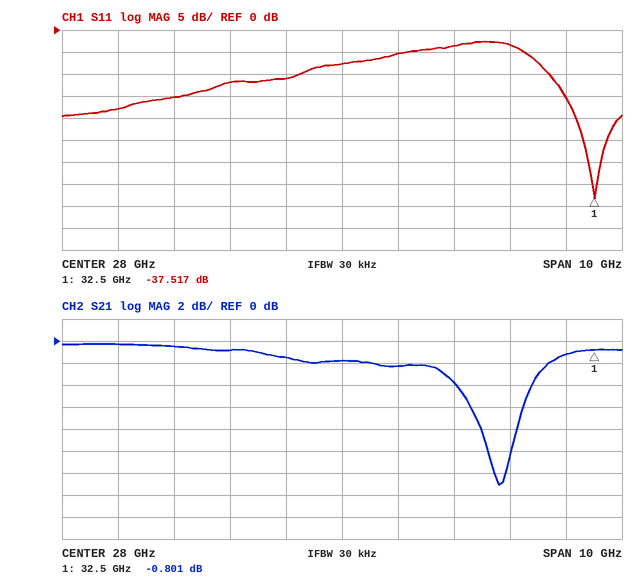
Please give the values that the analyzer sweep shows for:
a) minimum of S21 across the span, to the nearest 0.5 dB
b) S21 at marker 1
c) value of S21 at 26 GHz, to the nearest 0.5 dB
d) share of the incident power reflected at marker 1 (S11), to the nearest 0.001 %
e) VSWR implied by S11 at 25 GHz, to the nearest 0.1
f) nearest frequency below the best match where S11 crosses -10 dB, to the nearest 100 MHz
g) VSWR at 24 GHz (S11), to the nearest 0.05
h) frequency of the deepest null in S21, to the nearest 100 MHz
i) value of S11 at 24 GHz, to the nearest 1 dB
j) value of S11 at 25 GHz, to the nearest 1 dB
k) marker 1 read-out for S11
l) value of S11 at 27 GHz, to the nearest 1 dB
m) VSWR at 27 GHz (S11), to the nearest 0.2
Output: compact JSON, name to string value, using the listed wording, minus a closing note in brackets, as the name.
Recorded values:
{"minimum of S21 across the span, to the nearest 0.5 dB": "-13.0 dB", "S21 at marker 1": "-0.801 dB", "value of S21 at 26 GHz, to the nearest 0.5 dB": "-1.0 dB", "share of the incident power reflected at marker 1 (S11), to the nearest 0.001 %": "0.018 %", "VSWR implied by S11 at 25 GHz, to the nearest 0.1": "1.4", "nearest frequency below the best match where S11 crosses -10 dB, to the nearest 100 MHz": "31.7 GHz", "VSWR at 24 GHz (S11), to the nearest 0.05": "1.30", "frequency of the deepest null in S21, to the nearest 100 MHz": "30.8 GHz", "value of S11 at 24 GHz, to the nearest 1 dB": "-18 dB", "value of S11 at 25 GHz, to the nearest 1 dB": "-15 dB", "marker 1 read-out for S11": "-37.517 dB", "value of S11 at 27 GHz, to the nearest 1 dB": "-11 dB", "VSWR at 27 GHz (S11), to the nearest 0.2": "1.8"}
